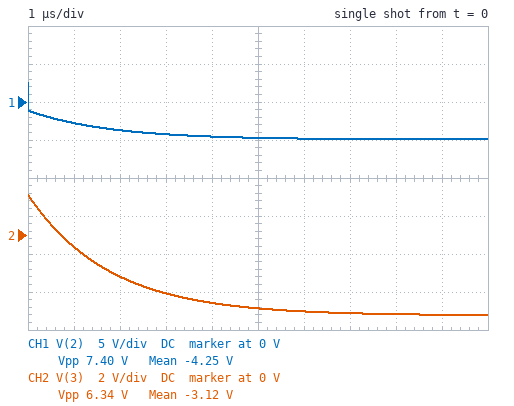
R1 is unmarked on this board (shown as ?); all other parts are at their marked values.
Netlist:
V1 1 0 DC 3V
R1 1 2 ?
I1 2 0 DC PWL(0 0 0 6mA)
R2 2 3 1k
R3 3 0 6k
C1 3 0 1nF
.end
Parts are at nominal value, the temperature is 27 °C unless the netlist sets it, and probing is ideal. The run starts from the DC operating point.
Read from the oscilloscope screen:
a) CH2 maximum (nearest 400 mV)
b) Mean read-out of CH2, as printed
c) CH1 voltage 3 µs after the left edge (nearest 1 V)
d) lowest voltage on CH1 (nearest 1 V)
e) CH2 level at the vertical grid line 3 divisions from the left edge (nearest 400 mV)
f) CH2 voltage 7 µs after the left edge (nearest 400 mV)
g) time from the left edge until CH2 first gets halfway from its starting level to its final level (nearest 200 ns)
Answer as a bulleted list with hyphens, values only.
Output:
- 2.0 V
- -3.12 V
- -4 V
- -5 V
- -3.2 V
- -4.0 V
- 1.2 µs
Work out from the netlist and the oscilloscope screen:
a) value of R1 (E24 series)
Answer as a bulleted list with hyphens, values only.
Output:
- 1.5 kΩ
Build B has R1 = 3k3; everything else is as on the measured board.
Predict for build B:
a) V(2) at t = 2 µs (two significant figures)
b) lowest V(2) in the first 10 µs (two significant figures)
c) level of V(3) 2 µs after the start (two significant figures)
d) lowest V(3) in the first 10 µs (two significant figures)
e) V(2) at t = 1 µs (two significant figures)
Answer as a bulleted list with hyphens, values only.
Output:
- -7.4 V
- -11 V
- -4.6 V
- -9.6 V
- -5.5 V
